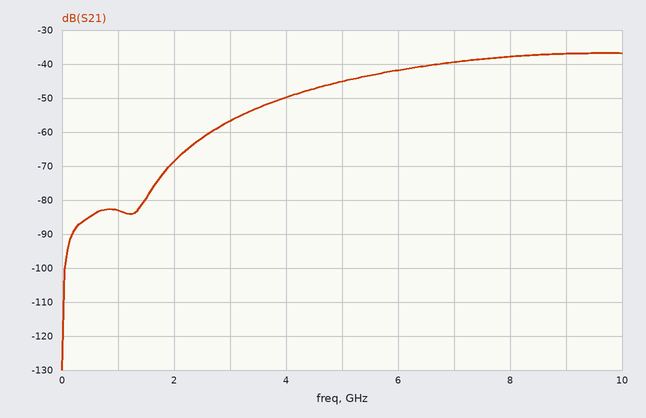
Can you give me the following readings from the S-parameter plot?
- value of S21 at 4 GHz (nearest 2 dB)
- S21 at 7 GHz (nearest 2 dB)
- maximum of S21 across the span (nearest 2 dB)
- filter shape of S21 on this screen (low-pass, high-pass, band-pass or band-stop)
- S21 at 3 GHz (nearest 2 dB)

-50 dB
-40 dB
-36 dB
high-pass
-56 dB
